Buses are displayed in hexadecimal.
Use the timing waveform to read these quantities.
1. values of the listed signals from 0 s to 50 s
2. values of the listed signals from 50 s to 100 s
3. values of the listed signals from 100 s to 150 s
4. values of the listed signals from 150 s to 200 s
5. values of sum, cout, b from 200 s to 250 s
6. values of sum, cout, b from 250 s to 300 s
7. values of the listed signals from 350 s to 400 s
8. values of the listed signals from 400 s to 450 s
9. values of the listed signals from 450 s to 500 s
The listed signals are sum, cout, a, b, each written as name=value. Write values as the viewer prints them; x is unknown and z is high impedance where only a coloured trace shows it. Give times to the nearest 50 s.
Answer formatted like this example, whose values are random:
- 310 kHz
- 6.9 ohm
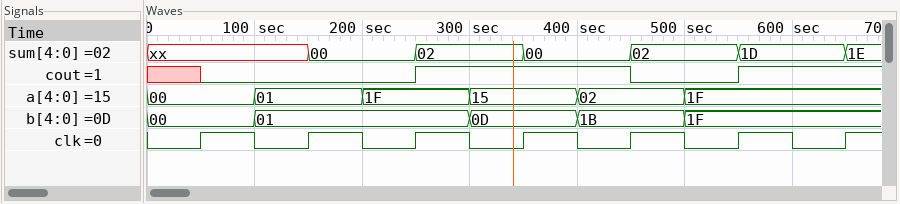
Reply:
- sum=xx, cout=x, a=00, b=00
- sum=xx, cout=0, a=00, b=00
- sum=xx, cout=0, a=01, b=01
- sum=00, cout=0, a=01, b=01
- sum=00, cout=0, b=01
- sum=02, cout=1, b=01
- sum=00, cout=1, a=15, b=0D
- sum=00, cout=1, a=02, b=1B
- sum=02, cout=0, a=02, b=1B
